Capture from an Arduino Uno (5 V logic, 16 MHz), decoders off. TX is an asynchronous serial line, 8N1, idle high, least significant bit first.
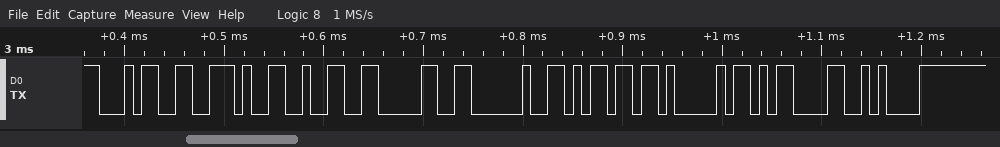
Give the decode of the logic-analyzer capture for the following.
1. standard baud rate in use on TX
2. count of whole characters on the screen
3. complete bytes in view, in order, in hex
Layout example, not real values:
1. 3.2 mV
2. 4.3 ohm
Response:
1. 115200 baud
2. 9
3. 0x34 0x2E 0x32 0x30 0x20 0x6D 0x41 0x0D 0x0A
